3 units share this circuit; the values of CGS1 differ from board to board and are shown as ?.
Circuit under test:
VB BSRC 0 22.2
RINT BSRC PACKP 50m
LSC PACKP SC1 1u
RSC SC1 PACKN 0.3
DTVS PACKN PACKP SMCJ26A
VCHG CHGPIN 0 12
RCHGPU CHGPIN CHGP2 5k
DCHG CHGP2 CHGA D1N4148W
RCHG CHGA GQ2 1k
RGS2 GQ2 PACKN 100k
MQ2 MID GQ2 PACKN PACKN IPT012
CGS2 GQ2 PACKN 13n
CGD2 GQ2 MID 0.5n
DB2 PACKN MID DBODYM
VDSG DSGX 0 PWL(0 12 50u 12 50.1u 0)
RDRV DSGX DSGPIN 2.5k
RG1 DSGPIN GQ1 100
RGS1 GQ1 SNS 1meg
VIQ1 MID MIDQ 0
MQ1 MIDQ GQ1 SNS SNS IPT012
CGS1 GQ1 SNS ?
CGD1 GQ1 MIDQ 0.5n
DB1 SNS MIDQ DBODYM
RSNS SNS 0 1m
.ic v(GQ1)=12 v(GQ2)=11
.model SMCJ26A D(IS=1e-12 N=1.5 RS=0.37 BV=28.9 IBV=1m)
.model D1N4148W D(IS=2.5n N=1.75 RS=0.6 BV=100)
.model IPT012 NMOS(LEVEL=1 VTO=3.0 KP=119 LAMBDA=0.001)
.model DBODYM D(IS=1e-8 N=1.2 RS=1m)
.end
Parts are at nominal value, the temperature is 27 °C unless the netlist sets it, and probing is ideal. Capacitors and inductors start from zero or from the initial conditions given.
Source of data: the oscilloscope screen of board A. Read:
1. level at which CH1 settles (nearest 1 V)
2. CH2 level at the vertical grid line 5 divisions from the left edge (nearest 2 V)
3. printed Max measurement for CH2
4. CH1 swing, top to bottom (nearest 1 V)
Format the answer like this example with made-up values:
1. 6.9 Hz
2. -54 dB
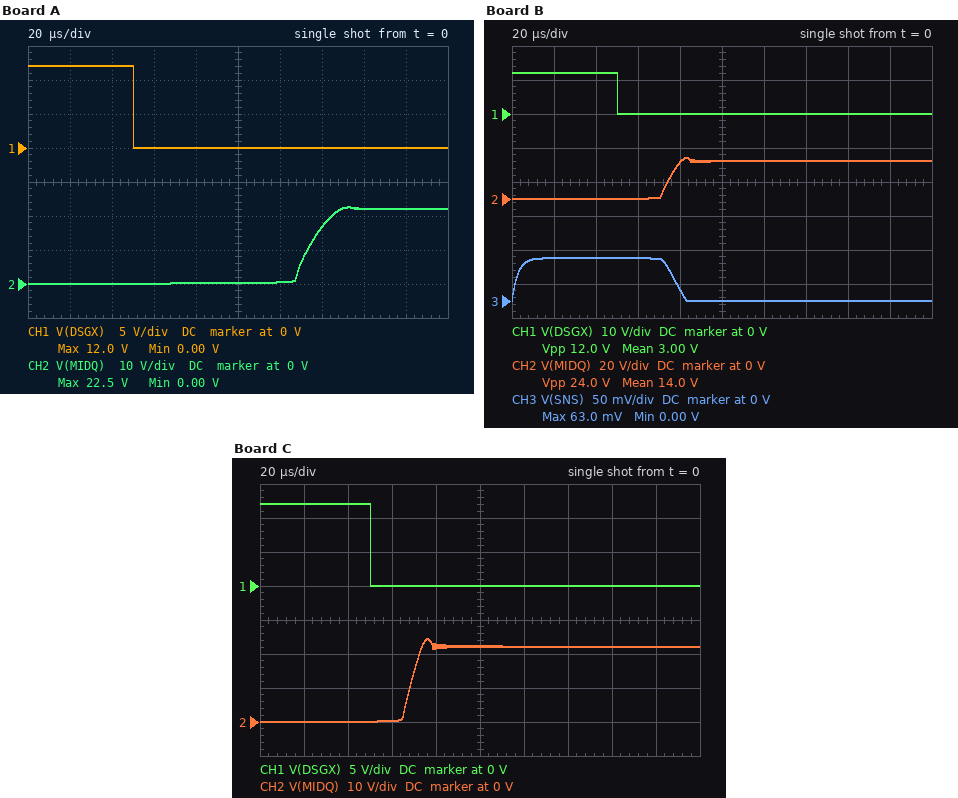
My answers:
1. 0 V
2. 0 V
3. 22.5 V
4. 12 V
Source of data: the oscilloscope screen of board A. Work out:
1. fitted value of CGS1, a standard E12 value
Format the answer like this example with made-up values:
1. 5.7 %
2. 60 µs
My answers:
1. 27 nF
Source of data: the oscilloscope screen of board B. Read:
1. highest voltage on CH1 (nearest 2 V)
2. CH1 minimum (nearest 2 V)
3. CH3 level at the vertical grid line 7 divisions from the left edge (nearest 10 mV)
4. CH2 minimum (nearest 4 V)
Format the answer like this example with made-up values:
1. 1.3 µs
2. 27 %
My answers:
1. 12 V
2. 0 V
3. 0 V
4. 0 V
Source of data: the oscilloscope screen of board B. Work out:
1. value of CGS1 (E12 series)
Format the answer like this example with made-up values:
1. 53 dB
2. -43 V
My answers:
1. 6.8 nF
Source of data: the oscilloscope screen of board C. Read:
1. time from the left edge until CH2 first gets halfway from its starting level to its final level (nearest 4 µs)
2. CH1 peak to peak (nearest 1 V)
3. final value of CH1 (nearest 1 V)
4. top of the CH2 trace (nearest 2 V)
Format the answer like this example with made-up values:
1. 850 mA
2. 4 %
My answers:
1. 68 µs
2. 12 V
3. 0 V
4. 24 V
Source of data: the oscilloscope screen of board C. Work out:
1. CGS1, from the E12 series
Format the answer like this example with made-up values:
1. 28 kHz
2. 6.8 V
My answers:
1. 4.7 nF
